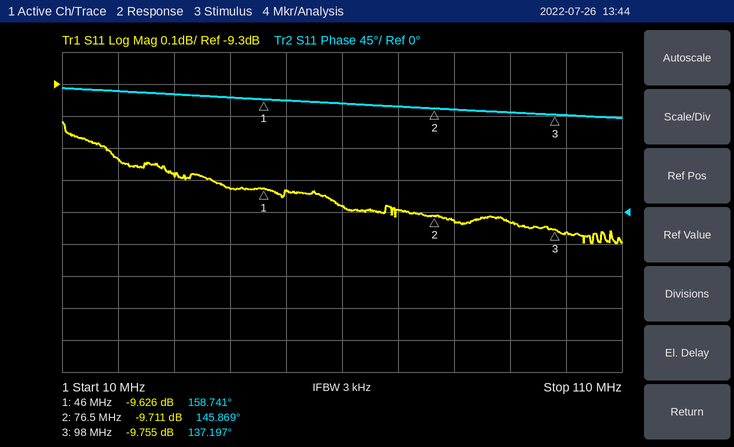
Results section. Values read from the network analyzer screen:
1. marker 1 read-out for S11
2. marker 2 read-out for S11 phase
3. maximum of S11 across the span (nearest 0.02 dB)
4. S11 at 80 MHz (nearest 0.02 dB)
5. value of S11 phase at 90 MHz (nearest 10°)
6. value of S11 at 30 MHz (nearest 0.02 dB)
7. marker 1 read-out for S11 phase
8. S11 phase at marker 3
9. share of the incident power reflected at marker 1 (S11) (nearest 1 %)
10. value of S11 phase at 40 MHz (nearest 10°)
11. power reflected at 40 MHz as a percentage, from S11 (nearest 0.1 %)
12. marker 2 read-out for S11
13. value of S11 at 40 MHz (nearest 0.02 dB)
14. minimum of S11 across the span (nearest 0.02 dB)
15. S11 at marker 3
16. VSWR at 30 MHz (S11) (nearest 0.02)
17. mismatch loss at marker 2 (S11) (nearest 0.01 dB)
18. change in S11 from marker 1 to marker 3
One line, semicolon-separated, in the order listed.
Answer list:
-9.626 dB; 145.869°; -9.42 dB; -9.72 dB; 140°; -9.58 dB; 158.741°; 137.197°; 11 %; 160°; 10.9 %; -9.711 dB; -9.62 dB; -9.80 dB; -9.755 dB; 2.00; 0.49 dB; -0.129 dB
